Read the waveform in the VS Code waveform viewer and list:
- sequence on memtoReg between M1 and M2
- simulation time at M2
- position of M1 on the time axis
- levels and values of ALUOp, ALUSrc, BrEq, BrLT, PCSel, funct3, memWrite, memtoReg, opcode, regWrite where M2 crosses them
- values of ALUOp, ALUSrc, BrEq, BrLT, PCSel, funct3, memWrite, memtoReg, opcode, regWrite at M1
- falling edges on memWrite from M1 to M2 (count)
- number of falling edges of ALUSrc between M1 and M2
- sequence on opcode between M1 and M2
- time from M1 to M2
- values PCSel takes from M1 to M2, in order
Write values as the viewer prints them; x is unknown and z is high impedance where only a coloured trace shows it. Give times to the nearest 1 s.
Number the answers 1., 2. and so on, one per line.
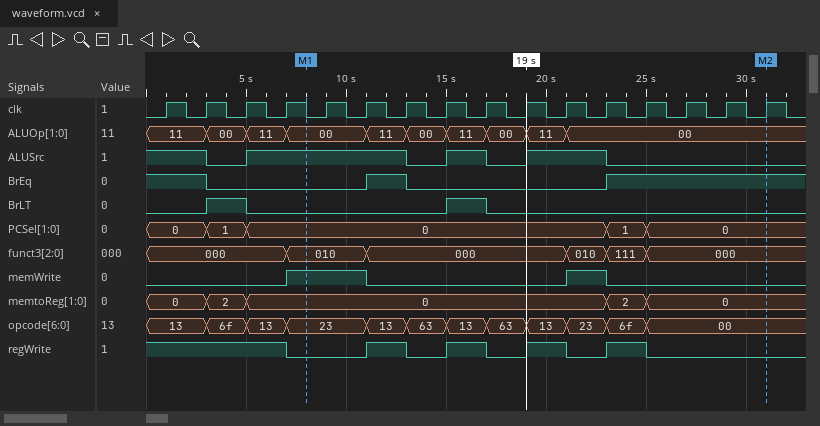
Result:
1. 0, 2, 0
2. 31 s
3. 8 s
4. ALUOp=00, ALUSrc=0, BrEq=1, BrLT=0, PCSel=0, funct3=000, memWrite=0, memtoReg=0, opcode=00, regWrite=0
5. ALUOp=00, ALUSrc=1, BrEq=0, BrLT=0, PCSel=0, funct3=010, memWrite=1, memtoReg=0, opcode=23, regWrite=0
6. 2
7. 3
8. 23, 13, 63, 13, 63, 13, 23, 6f, 00
9. 23 s
10. 0, 1, 0
